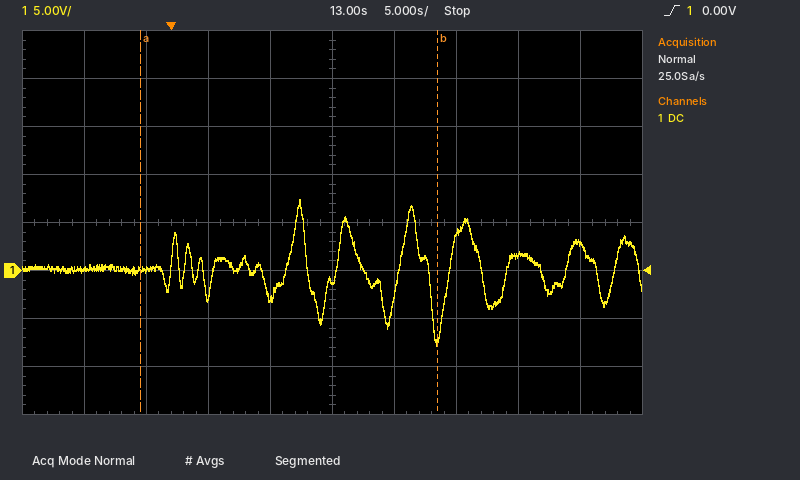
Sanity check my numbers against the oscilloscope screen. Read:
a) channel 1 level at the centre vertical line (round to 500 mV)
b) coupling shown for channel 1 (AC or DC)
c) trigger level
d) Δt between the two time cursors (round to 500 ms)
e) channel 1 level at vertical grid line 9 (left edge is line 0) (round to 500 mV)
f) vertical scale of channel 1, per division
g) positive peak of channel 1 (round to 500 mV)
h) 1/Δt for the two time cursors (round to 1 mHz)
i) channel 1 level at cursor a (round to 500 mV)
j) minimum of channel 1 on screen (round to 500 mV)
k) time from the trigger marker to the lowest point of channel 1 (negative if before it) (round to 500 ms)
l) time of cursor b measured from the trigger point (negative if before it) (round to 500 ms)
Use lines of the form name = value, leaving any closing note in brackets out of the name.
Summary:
channel 1 level at the centre vertical line = -1.0 V
coupling shown for channel 1 = DC
trigger level = 0.00 V
Δt between the two time cursors = 24.0 s
channel 1 level at vertical grid line 9 (left edge is line 0) = 3.0 V
vertical scale of channel 1, per division = 5 V
positive peak of channel 1 = 7.5 V
1/Δt for the two time cursors = 42 mHz
channel 1 level at cursor a = 0.0 V
minimum of channel 1 on screen = -8.0 V
time from the trigger marker to the lowest point of channel 1 (negative if before it) = +21.5 s
time of cursor b measured from the trigger point (negative if before it) = +21.5 s
